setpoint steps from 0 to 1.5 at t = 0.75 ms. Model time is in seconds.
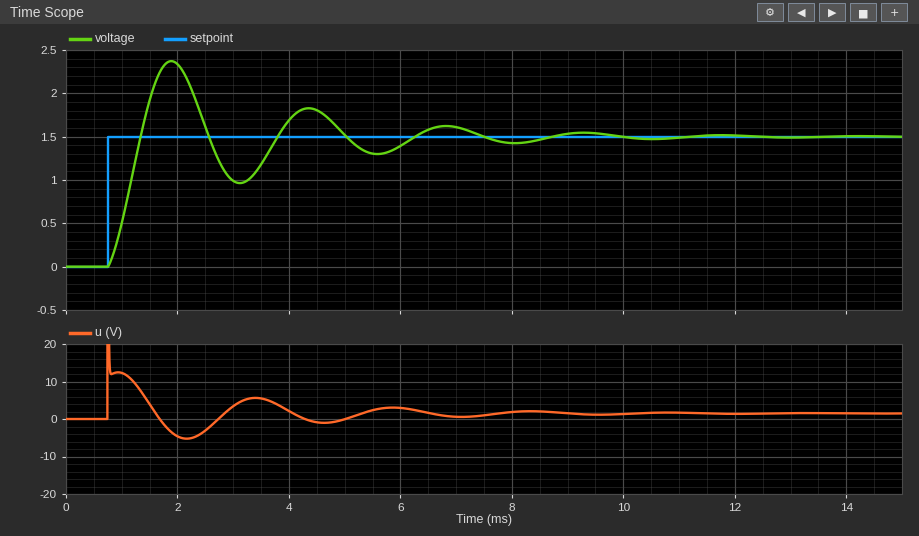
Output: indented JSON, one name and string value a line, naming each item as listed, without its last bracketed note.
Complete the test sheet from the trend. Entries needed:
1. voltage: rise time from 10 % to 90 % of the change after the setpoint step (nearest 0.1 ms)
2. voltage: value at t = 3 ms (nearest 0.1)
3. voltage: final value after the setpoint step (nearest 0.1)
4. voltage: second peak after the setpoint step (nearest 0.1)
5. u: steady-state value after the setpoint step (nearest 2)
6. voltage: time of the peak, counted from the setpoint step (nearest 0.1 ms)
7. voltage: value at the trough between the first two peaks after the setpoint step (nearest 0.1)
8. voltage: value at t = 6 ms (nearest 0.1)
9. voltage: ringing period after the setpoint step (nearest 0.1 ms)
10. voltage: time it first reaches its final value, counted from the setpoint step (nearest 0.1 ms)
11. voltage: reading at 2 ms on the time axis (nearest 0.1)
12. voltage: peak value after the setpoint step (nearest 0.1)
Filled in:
{
  "voltage: rise time from 10 % to 90 % of the change after the setpoint step": "0.4 ms",
  "voltage: value at t = 3 ms": "1.0",
  "voltage: final value after the setpoint step": "1.5",
  "voltage: second peak after the setpoint step": "1.8",
  "u: steady-state value after the setpoint step": "2",
  "voltage: time of the peak, counted from the setpoint step": "1.1 ms",
  "voltage: value at the trough between the first two peaks after the setpoint step": "1.0",
  "voltage: value at t = 6 ms": "1.4",
  "voltage: ringing period after the setpoint step": "2.5 ms",
  "voltage: time it first reaches its final value, counted from the setpoint step": "0.6 ms",
  "voltage: reading at 2 ms on the time axis": "2.3",
  "voltage: peak value after the setpoint step": "2.4"
}
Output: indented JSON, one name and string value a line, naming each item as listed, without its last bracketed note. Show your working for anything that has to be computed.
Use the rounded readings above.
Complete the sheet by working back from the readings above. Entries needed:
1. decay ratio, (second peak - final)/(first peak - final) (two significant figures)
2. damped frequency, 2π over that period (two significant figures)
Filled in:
{
  "decay ratio, (second peak - final)/(first peak - final)": "(1.8 - 1.5) / (2.4 - 1.5) = 0.33",
  "damped frequency, 2π over that period": "2π / 2.5 = 2.5 rad/ms"
}
